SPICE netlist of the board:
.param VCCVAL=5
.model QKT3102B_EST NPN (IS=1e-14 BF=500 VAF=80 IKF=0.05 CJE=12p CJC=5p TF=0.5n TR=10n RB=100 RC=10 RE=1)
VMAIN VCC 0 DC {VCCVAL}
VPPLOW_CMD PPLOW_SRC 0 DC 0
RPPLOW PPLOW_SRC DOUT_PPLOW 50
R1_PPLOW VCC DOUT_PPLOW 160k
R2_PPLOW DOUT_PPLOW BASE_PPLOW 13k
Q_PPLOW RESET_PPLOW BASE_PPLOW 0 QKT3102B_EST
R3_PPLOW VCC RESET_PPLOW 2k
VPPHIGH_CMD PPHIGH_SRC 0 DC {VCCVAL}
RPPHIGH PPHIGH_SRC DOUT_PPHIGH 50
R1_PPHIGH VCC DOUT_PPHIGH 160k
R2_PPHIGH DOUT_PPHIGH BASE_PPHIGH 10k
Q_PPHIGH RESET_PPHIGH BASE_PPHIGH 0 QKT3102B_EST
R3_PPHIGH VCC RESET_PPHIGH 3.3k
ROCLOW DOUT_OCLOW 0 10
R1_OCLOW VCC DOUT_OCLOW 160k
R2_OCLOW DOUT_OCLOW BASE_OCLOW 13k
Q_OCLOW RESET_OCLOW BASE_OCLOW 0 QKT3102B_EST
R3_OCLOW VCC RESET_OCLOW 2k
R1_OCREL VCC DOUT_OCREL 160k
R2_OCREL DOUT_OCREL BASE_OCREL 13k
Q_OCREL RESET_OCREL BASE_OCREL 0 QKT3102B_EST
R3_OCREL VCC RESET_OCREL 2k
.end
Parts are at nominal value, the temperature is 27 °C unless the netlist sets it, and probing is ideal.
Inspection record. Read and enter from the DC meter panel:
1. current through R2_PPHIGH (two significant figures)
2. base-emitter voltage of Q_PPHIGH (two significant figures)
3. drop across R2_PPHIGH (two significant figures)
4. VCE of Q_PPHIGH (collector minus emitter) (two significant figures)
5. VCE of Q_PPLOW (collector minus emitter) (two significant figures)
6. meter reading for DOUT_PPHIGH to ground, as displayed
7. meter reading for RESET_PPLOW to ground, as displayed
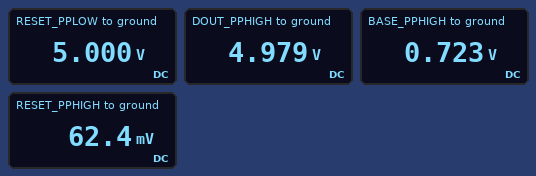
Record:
430 µA
720 mV
4.3 V
62 mV
5.0 V
4.979 V
5.000 V
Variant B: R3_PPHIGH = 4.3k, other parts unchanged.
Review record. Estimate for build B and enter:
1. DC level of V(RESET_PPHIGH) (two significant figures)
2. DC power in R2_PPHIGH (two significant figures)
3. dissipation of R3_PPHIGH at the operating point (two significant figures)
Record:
54 mV
1.8 mW
5.7 mW
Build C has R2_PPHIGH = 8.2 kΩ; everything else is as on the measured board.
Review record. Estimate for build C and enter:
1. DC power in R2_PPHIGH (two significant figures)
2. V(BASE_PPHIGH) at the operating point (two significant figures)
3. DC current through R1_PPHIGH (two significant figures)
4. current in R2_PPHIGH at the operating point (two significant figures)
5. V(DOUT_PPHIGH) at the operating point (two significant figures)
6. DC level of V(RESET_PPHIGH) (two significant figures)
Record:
2.2 mW
730 mV
160 nA
520 µA
5.0 V
59 mV
